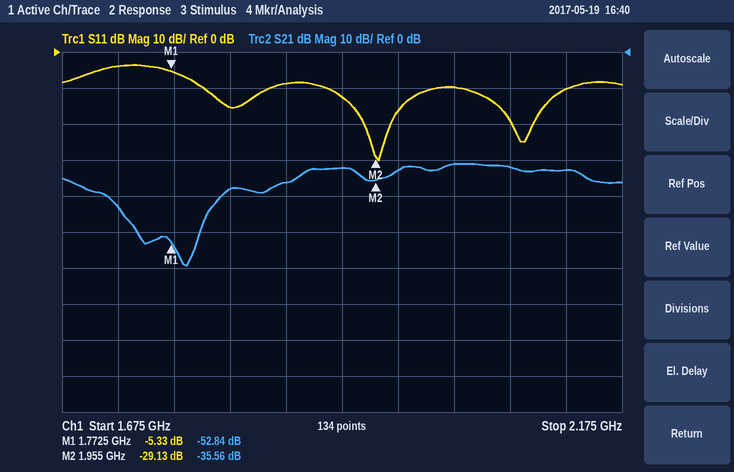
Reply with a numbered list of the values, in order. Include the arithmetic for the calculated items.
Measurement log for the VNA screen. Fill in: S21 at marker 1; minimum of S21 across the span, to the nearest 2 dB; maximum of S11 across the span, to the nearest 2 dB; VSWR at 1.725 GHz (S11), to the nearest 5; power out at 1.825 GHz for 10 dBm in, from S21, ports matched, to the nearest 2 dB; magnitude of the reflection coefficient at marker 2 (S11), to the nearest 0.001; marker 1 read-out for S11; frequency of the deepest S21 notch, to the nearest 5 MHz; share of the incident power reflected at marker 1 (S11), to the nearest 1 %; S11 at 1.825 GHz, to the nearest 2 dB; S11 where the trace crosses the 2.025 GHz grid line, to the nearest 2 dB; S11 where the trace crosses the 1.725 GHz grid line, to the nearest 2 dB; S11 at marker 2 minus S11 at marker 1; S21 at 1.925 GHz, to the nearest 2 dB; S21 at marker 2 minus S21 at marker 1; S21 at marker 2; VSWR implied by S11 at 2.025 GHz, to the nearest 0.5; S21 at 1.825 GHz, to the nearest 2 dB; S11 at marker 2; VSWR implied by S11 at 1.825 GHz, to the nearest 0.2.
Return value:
1. -52.84 dB
2. -60 dB
3. -4 dB
4. |Γ| = 10^(-4/20) = 0.6310; VSWR = (1 + 0.6310)/(1 − 0.6310) ≈ 4.42, so 5 to the nearest 5
5. 10 dBm + (-38 dB) = -28 dBm
6. 10^(-29.13/20) ≈ 0.035
7. -5.33 dB
8. 1.785 GHz
9. 10^(-5.33/10) ≈ 29 %
10. -16 dB
11. -10 dB
12. -4 dB
13. -29.13 − (-5.33) = -23.80 dB
14. -32 dB
15. -35.56 − (-52.84) = 17.28 dB
16. -35.56 dB
17. |Γ| = 10^(-10/20) = 0.3162; VSWR = (1 + 0.3162)/(1 − 0.3162) ≈ 1.92, so 2.0 to the nearest 0.5
18. -38 dB
19. -29.13 dB
20. |Γ| = 10^(-16/20) = 0.1585; VSWR = (1 + 0.1585)/(1 − 0.1585) ≈ 1.4
